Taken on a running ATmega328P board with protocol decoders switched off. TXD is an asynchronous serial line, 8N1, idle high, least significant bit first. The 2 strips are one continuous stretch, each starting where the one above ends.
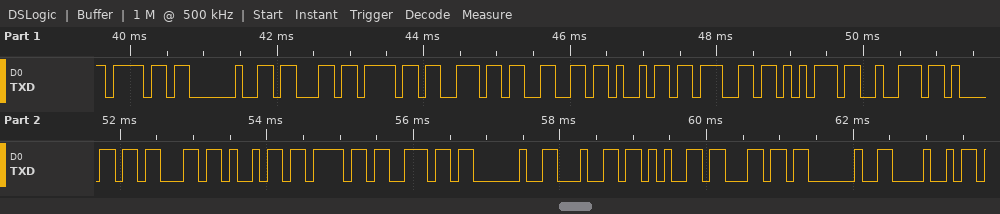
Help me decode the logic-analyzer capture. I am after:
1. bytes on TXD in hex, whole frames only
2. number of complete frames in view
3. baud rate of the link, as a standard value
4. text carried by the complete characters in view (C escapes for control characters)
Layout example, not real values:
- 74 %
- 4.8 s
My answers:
- 0x6F 0x20 0x63 0x6F 0x6E 0x66 0x69 0x67 0x75 0x72 0x61 0x63 0x69 0x6F 0x6E 0x20 0x64 0x65 0x6C 0x20 0x48
- 21
- 9600 baud
- "o configuracion del H"
